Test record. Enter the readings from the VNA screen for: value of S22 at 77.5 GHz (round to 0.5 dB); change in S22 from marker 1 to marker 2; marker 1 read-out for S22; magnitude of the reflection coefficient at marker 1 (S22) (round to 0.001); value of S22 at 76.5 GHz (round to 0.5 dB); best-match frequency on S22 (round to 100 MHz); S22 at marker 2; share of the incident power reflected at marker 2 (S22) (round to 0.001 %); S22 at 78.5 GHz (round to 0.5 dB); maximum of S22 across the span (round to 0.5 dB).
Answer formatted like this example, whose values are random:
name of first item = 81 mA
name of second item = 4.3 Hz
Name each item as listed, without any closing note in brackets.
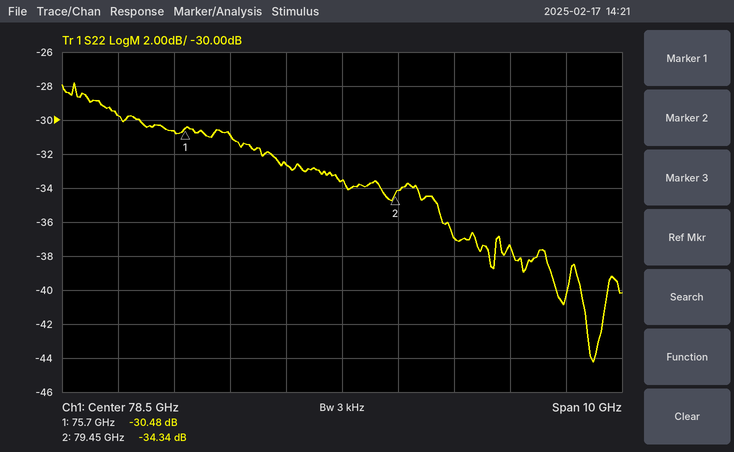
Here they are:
value of S22 at 77.5 GHz = -32.5 dB
change in S22 from marker 1 to marker 2 = -3.86 dB
marker 1 read-out for S22 = -30.48 dB
magnitude of the reflection coefficient at marker 1 (S22) = 0.030
value of S22 at 76.5 GHz = -31.0 dB
best-match frequency on S22 = 83.0 GHz
S22 at marker 2 = -34.34 dB
share of the incident power reflected at marker 2 (S22) = 0.037 %
S22 at 78.5 GHz = -33.5 dB
maximum of S22 across the span = -28.0 dB
